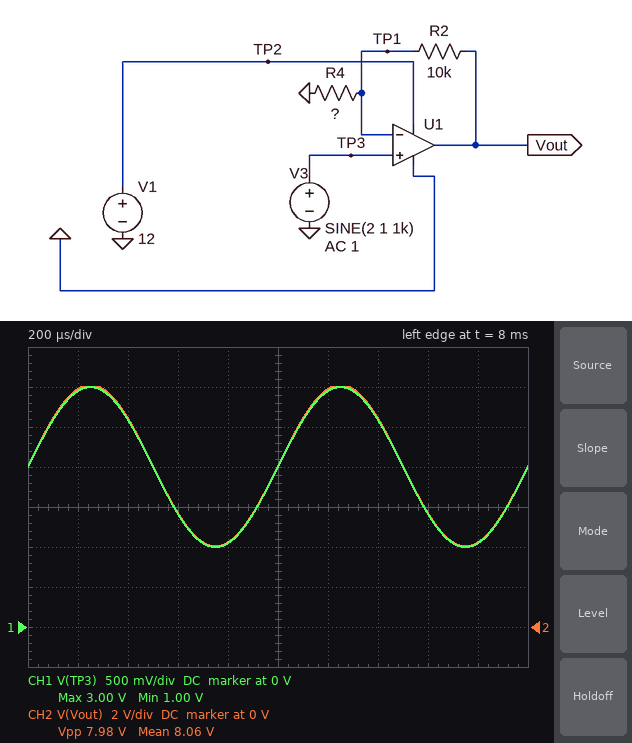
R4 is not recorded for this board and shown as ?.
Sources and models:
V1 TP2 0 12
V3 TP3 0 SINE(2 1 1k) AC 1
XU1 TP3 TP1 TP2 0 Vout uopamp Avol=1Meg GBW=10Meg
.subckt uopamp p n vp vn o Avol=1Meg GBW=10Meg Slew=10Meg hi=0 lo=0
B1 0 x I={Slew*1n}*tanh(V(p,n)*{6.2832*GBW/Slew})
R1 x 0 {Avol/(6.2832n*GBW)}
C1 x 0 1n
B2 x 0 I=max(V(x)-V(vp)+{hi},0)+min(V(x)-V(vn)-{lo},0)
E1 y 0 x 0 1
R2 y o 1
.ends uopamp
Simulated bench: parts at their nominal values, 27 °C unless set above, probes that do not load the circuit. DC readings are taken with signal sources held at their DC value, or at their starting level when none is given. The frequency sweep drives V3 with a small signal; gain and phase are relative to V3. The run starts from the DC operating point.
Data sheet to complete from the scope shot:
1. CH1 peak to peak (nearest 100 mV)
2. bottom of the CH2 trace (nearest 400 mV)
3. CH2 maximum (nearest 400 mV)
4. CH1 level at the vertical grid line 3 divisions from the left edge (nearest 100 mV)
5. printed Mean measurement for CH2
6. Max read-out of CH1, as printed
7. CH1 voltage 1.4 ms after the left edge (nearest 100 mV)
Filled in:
2.0 V
4.0 V
12.0 V
1.4 V
8.06 V
3.00 V
2.6 V
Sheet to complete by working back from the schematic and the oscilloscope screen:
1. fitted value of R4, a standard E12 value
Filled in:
3.3 kΩ
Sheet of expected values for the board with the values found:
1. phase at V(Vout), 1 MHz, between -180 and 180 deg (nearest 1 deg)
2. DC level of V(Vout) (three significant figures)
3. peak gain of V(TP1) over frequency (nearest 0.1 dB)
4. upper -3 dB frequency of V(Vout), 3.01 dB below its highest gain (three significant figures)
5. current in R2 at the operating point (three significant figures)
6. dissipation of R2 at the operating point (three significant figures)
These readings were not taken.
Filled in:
-22 deg
8.06 V
0 dB
2.48 MHz
606 µA
3.67 mW
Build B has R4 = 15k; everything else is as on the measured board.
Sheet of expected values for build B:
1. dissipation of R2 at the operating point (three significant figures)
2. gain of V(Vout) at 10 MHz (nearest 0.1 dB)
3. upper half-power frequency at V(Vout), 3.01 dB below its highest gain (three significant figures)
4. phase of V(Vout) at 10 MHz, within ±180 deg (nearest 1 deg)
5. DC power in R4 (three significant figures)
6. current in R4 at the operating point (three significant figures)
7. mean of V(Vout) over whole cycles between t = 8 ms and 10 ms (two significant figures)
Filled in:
178 µW
-1.3 dB
6.00 MHz
-59 deg
267 µW
133 µA
3.3 V
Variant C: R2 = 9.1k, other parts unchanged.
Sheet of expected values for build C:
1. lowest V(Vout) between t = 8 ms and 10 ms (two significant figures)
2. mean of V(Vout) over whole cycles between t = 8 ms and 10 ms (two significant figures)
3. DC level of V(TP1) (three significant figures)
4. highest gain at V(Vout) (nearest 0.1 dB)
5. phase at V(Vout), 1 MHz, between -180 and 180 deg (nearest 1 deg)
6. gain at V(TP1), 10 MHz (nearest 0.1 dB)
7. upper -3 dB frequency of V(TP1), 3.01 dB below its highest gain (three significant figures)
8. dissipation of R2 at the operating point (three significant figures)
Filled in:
3.8 V
7.5 V
2.00 V
11.5 dB
-21 deg
-11.8 dB
2.66 MHz
3.34 mW
